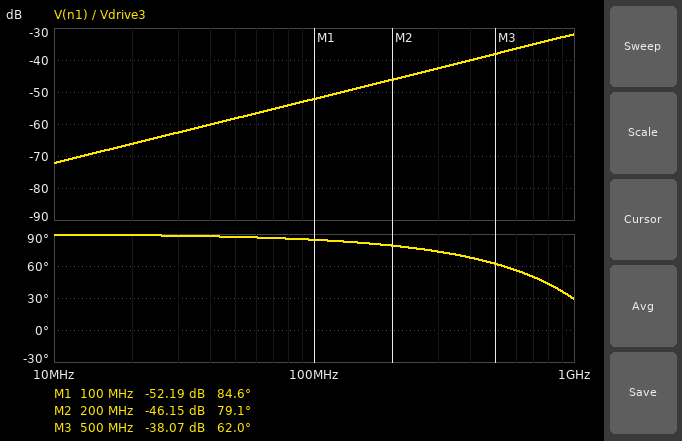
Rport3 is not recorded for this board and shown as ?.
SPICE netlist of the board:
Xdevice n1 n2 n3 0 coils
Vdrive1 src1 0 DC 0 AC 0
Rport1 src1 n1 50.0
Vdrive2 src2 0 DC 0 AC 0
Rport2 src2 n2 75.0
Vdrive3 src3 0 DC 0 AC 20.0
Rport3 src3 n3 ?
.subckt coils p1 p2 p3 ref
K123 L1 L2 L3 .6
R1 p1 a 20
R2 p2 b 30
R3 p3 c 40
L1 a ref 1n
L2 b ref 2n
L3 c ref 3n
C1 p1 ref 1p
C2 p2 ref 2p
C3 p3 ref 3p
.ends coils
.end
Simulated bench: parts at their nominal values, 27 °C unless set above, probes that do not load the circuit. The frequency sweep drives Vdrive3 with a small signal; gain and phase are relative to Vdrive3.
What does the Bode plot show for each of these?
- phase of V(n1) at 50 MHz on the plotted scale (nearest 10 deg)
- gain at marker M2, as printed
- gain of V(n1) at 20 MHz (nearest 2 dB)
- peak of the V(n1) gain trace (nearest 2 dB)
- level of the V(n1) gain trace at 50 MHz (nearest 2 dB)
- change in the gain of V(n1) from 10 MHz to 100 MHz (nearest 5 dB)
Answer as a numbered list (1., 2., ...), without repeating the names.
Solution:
1. 90 deg
2. -46.15 dB
3. -66 dB
4. -32 dB
5. -58 dB
6. 20 dB
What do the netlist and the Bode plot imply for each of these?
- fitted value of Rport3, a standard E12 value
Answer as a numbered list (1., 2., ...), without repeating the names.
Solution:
1. 150 Ω
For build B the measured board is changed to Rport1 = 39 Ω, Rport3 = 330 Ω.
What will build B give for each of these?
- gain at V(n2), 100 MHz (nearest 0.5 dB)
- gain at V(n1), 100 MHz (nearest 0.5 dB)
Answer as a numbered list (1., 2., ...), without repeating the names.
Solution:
1. -55.0 dB
2. -58.5 dB
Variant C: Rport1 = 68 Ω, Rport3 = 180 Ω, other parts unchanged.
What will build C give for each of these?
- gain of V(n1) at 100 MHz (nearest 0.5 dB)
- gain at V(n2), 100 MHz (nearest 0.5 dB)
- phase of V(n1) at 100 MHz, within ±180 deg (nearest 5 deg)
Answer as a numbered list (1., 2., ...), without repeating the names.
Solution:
1. -53.0 dB
2. -50.5 dB
3. 85 deg
